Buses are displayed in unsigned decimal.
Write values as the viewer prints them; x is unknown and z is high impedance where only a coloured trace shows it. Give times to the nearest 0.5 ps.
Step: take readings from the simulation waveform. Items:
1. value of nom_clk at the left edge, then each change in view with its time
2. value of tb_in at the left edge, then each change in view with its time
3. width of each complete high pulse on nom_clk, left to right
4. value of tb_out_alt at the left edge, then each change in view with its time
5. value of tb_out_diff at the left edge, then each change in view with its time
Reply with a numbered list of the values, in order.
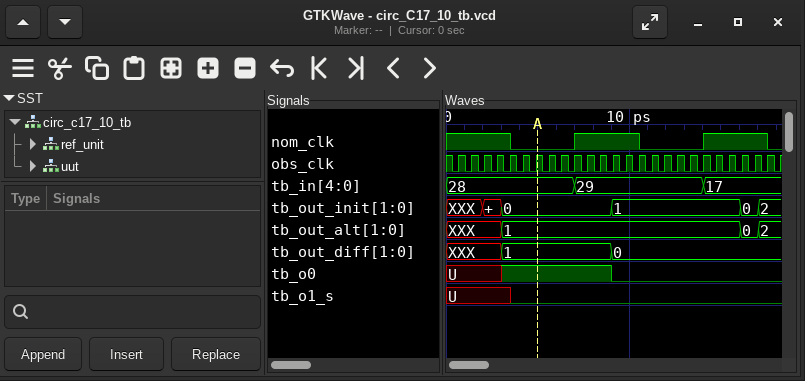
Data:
1. 1, 0 at 3.5 ps, 1 at 7 ps, 0 at 10.5 ps, 1 at 14 ps, 0 at 17.5 ps
2. 28, 29 at 7 ps, 17 at 14 ps
3. 3.5 ps, 3.5 ps
4. XXX, 1 at 3 ps, 0 at 16 ps, 2 at 17 ps
5. XXX, 1 at 3 ps, 0 at 9 ps
